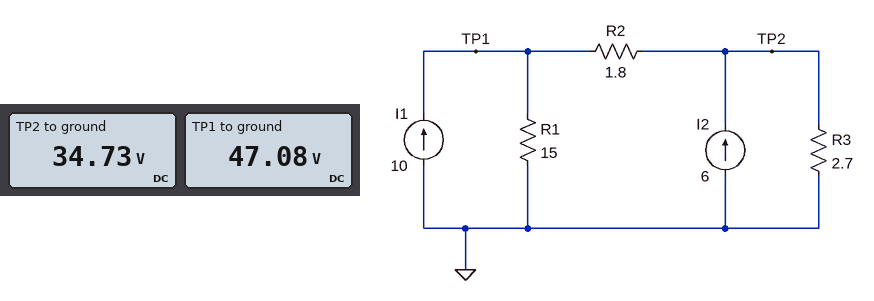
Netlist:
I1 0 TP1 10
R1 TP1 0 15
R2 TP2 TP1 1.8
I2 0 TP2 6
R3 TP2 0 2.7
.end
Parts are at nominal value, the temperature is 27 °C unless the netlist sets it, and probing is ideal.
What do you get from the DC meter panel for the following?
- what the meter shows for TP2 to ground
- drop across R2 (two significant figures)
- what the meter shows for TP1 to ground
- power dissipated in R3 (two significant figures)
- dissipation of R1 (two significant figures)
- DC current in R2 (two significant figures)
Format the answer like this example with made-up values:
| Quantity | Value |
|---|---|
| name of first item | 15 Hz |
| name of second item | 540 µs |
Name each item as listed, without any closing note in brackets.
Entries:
| Quantity | Value |
|---|---|
| what the meter shows for TP2 to ground | 34.73 V |
| drop across R2 | 12 V |
| what the meter shows for TP1 to ground | 47.08 V |
| power dissipated in R3 | 450 W |
| dissipation of R1 | 150 W |
| DC current in R2 | 6.9 A |
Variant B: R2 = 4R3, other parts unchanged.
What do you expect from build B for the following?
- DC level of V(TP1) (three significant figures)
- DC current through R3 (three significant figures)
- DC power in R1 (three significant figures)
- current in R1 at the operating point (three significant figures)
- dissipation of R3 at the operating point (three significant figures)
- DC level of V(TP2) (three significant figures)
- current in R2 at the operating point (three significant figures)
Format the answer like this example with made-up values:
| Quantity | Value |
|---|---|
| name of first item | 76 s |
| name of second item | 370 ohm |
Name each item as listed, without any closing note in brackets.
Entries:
| Quantity | Value |
|---|---|
| DC level of V(TP1) | 58.8 V |
| DC current through R3 | 12.1 A |
| DC power in R1 | 230 W |
| current in R1 at the operating point | 3.92 A |
| dissipation of R3 at the operating point | 394 W |
| DC level of V(TP2) | 32.6 V |
| current in R2 at the operating point | 6.08 A |
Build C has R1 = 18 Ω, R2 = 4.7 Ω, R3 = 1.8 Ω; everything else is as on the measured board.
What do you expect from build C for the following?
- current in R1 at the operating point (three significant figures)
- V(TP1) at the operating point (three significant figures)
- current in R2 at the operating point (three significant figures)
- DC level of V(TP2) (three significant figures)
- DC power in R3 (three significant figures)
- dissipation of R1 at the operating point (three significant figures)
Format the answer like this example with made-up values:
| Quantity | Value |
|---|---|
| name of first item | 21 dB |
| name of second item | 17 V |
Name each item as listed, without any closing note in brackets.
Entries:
| Quantity | Value |
|---|---|
| current in R1 at the operating point | 3.09 A |
| V(TP1) at the operating point | 55.7 V |
| current in R2 at the operating point | 6.91 A |
| DC level of V(TP2) | 23.2 V |
| DC power in R3 | 300 W |
| dissipation of R1 at the operating point | 172 W |
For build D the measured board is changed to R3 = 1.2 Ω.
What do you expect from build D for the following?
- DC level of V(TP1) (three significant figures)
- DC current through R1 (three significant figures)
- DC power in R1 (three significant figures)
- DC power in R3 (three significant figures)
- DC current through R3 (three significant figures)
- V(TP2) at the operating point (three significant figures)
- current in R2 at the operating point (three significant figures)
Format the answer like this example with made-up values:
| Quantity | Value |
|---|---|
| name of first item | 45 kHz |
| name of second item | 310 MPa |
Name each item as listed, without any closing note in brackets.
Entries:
| Quantity | Value |
|---|---|
| DC level of V(TP1) | 31.0 V |
| DC current through R1 | 2.07 A |
| DC power in R1 | 64.1 W |
| DC power in R3 | 233 W |
| DC current through R3 | 13.9 A |
| V(TP2) at the operating point | 16.7 V |
| current in R2 at the operating point | 7.93 A |
